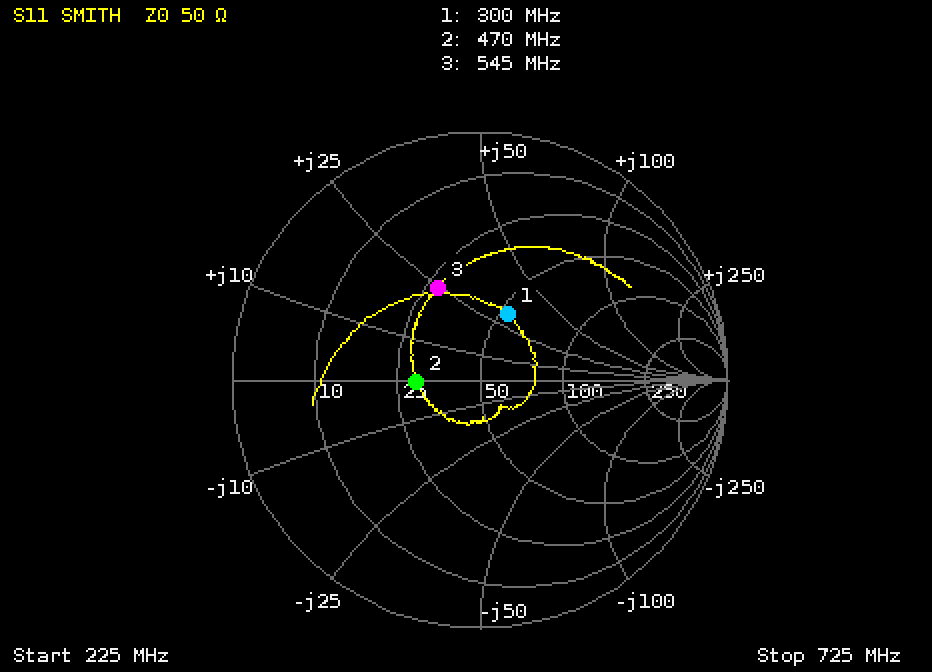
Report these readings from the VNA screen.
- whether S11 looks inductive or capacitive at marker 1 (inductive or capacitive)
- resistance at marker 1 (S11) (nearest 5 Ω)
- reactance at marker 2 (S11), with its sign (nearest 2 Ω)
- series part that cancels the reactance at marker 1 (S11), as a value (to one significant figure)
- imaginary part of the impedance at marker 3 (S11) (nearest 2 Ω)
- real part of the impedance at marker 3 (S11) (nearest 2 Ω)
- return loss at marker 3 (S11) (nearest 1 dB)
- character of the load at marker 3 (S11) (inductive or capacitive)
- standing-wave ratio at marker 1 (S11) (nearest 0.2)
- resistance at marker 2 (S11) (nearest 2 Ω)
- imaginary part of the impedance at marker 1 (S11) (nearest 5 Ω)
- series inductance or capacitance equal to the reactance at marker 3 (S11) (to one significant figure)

inductive
55 Ω
0 Ω
20 pF
+24 Ω
28 Ω
8 dB
inductive
1.8
30 Ω
+30 Ω
7 nH
